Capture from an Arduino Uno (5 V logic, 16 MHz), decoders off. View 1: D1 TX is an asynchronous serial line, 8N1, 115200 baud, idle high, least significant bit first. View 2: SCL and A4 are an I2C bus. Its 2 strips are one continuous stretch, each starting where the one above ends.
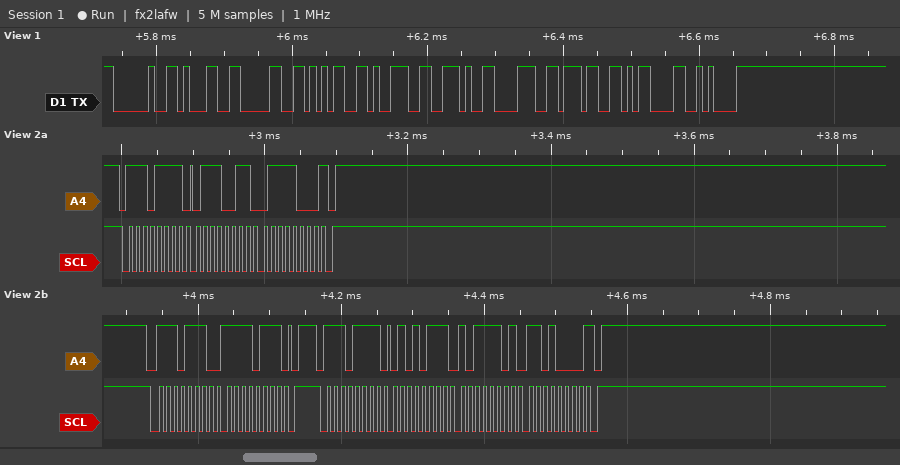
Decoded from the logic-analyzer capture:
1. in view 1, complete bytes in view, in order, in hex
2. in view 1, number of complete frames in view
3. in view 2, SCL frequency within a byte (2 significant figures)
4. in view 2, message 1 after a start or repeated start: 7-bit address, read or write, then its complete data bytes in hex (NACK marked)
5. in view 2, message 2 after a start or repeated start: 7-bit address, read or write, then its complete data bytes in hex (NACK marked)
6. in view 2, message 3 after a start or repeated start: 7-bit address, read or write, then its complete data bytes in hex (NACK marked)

20 31 30 35 39 2E 38 37 0D 0A
10
100 kHz
0x77 read: 73 78 NACK
0x77 write: F7
0x77 read: 57 BD D0 NACK
